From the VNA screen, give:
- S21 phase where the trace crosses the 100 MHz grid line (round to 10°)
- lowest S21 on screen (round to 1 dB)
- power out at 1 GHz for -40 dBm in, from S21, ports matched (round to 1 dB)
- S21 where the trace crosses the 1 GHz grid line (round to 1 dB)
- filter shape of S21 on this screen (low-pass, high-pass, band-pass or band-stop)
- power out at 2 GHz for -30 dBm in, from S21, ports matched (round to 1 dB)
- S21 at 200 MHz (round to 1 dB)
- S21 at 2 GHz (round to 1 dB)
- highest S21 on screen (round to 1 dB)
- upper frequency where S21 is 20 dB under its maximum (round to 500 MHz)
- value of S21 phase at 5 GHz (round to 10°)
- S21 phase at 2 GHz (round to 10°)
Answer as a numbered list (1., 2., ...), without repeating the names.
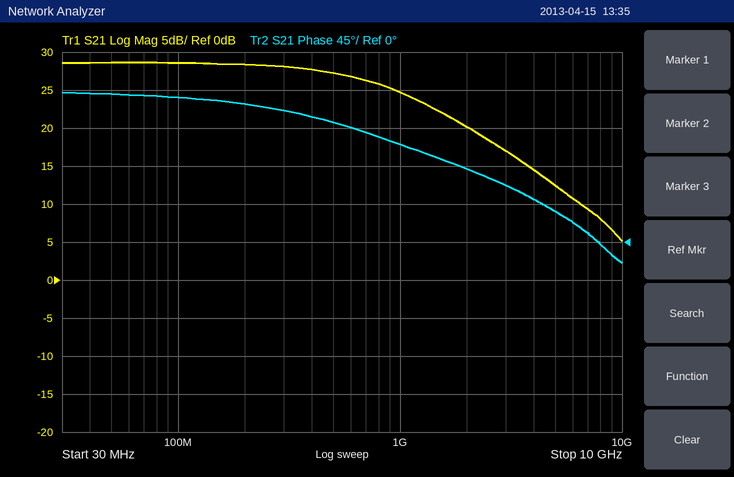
1. 170°
2. 5 dB
3. -15 dBm
4. 25 dB
5. low-pass
6. -10 dBm
7. 28 dB
8. 20 dB
9. 29 dB
10. 7.5 GHz
11. 40°
12. 90°
